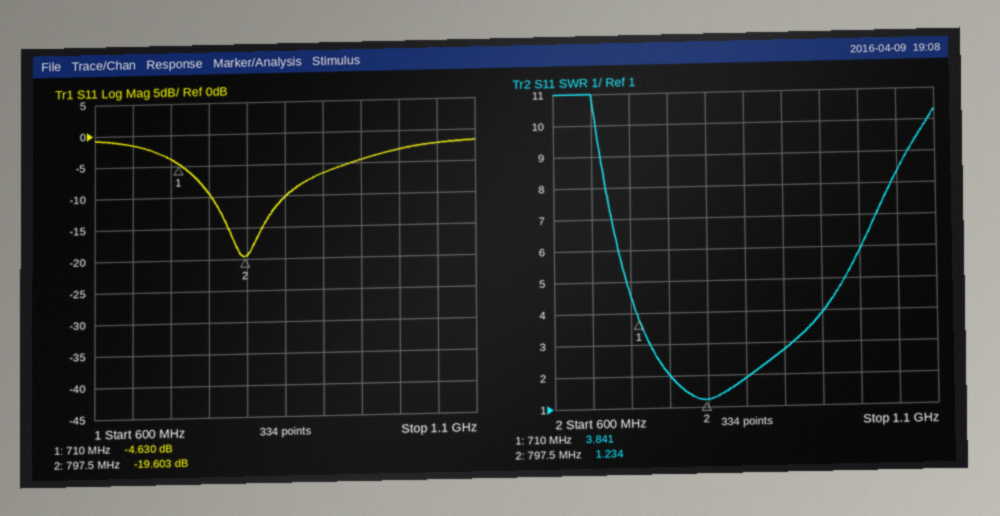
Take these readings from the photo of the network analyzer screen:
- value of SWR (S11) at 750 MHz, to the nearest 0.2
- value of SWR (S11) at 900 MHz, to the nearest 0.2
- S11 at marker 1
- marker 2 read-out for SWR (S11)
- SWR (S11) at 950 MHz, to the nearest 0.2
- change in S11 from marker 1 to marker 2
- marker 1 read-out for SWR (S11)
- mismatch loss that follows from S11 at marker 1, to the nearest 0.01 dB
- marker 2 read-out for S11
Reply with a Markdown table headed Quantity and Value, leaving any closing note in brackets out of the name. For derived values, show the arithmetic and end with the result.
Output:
| Quantity | Value |
|---|---|
| value of SWR (S11) at 750 MHz, to the nearest 0.2 | 2.0 |
| value of SWR (S11) at 900 MHz, to the nearest 0.2 | 2.8 |
| S11 at marker 1 | -4.630 dB |
| marker 2 read-out for SWR | 1.234 |
| SWR (S11) at 950 MHz, to the nearest 0.2 | 4.0 |
| change in S11 from marker 1 to marker 2 | -19.603 − (-4.63) = -14.973 dB |
| marker 1 read-out for SWR | 3.841 |
| mismatch loss that follows from S11 at marker 1, to the nearest 0.01 dB | −10 log10(1 − 10^(-4.63/10)) ≈ 1.83 dB |
| marker 2 read-out for S11 | -19.603 dB |
